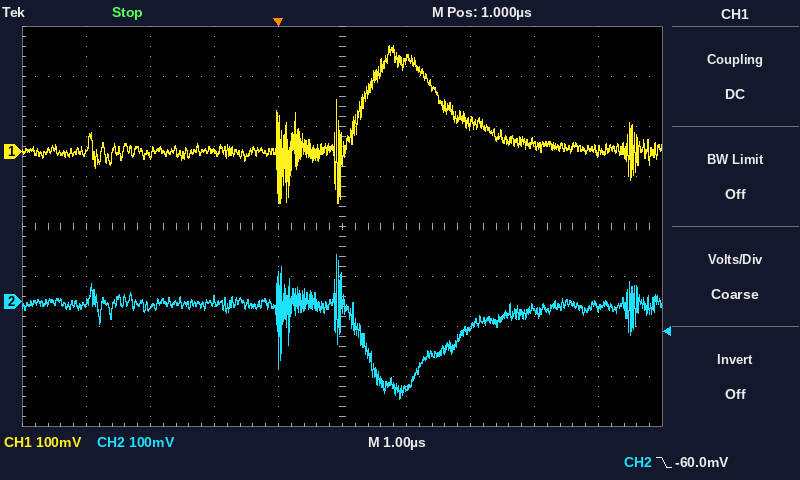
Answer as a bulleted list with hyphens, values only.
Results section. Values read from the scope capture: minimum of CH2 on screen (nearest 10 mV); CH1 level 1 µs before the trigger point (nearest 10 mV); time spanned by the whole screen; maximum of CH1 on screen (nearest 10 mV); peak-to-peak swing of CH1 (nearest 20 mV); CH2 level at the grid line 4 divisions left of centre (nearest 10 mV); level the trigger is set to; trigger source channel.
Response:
- -200 mV
- 0 mV
- 10 µs
- 210 mV
- 320 mV
- 0 mV
- -60.0 mV
- CH2
